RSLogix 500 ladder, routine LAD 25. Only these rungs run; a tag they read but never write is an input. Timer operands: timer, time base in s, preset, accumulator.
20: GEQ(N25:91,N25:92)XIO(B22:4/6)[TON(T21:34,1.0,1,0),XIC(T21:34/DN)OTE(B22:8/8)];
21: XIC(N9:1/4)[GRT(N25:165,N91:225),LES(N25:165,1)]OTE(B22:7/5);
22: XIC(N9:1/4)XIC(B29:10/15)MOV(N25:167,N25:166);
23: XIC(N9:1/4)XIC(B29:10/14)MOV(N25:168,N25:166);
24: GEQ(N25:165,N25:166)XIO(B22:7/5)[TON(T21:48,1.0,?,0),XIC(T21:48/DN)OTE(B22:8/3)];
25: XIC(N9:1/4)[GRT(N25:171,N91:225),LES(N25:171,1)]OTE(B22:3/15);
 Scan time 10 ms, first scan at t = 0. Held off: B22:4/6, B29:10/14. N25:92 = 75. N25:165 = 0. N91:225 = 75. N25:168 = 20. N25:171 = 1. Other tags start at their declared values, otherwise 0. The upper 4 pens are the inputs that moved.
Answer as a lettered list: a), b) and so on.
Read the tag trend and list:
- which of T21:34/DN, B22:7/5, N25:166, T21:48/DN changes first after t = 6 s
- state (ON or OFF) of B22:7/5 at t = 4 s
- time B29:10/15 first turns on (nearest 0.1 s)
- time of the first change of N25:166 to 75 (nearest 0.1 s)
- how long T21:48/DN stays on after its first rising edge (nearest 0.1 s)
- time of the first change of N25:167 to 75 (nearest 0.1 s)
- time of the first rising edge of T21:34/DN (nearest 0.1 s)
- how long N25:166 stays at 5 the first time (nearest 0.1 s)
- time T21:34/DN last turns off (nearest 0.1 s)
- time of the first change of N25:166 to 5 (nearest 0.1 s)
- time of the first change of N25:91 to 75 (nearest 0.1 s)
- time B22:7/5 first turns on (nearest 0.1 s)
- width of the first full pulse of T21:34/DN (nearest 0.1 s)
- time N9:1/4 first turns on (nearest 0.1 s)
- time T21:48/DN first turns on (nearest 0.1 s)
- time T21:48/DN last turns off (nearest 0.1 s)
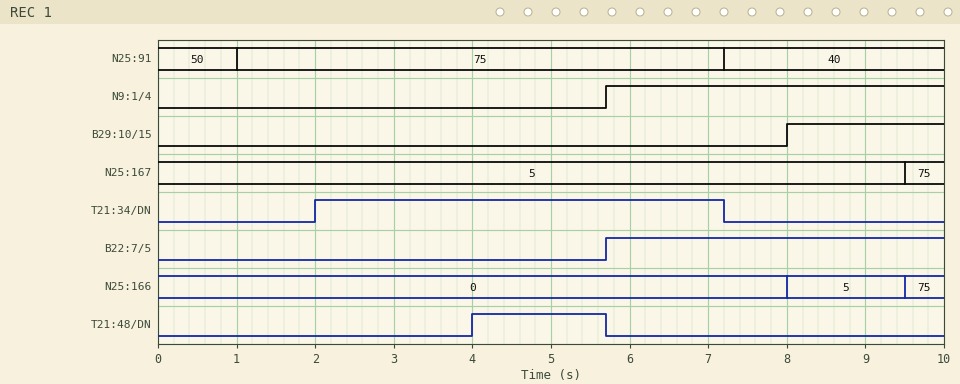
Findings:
a) T21:34/DN
b) OFF
c) 8.0 s
d) 9.5 s
e) 1.7 s
f) 9.5 s
g) 2.0 s
h) 1.5 s
i) 7.2 s
j) 8.0 s
k) 1.0 s
l) 5.7 s
m) 5.2 s
n) 5.7 s
o) 4.0 s
p) 5.7 s
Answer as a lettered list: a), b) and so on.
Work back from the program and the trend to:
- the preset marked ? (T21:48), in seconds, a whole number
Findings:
a) 4 s
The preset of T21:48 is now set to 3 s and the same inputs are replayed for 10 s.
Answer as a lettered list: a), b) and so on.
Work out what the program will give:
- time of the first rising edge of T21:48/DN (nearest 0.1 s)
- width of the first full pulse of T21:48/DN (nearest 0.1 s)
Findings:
a) 3.0 s
b) 2.7 s
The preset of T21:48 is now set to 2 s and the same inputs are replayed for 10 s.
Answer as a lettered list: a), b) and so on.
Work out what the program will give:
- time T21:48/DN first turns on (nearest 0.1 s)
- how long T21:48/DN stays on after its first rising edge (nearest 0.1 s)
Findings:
a) 2.0 s
b) 3.7 s
